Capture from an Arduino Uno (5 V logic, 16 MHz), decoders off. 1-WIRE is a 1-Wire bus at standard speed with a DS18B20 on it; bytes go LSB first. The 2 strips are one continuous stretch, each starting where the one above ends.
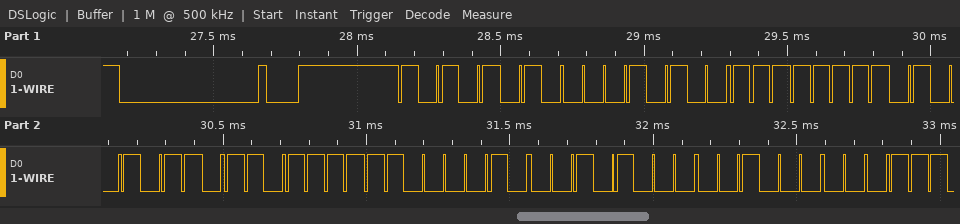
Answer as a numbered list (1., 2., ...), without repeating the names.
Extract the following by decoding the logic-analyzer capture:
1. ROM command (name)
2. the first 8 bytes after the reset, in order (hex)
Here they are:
1. Match ROM
2. 55 28 FF D2 F6 43 14 04
